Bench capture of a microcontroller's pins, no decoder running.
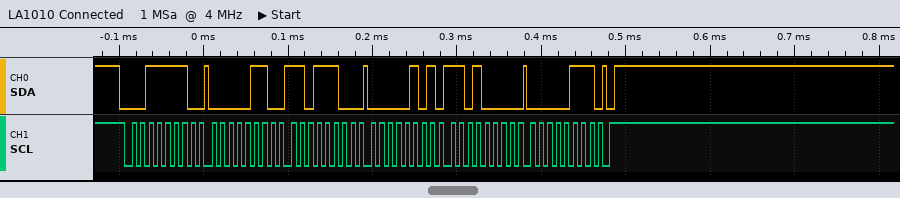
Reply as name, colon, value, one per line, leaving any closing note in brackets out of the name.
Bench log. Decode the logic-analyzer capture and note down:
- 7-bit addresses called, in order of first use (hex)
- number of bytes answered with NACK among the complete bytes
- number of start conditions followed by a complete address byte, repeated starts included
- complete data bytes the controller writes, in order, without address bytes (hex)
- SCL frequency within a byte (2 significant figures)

7-bit addresses called, in order of first use: 0x1F
number of bytes answered with NACK among the complete bytes: 0
number of start conditions followed by a complete address byte, repeated starts included: 1
complete data bytes the controller writes, in order, without address bytes: 06 DC 05 D0 07
SCL frequency within a byte: 100 kHz
